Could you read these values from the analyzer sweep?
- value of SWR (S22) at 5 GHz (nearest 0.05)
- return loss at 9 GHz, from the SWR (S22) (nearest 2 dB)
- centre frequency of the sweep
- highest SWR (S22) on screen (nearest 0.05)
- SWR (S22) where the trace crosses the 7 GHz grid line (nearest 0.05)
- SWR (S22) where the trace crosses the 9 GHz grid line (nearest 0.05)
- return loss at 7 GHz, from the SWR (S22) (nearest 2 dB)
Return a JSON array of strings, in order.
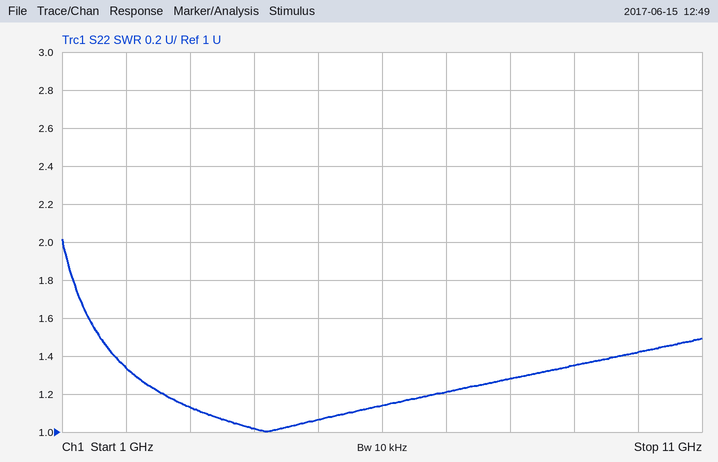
["1.05", "16 dB", "6 GHz", "2.00", "1.20", "1.35", "20 dB"]
